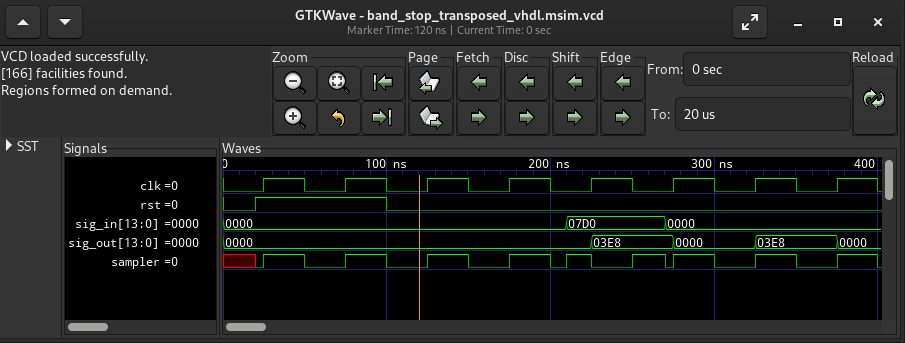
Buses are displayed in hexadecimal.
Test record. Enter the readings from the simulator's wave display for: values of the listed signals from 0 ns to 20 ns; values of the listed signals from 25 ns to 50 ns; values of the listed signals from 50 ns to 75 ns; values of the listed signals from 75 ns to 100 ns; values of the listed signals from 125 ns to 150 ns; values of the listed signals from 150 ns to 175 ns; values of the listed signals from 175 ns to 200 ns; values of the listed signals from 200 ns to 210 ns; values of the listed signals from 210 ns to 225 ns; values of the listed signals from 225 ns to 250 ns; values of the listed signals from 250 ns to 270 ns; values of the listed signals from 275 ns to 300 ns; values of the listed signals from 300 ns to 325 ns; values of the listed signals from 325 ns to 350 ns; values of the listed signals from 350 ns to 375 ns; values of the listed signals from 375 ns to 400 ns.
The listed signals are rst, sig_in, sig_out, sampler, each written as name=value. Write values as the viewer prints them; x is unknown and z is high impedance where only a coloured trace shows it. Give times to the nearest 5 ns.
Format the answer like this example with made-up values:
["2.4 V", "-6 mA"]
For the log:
["rst=0, sig_in=0000, sig_out=0000, sampler=x", "rst=1, sig_in=0000, sig_out=0000, sampler=1", "rst=1, sig_in=0000, sig_out=0000, sampler=0", "rst=1, sig_in=0000, sig_out=0000, sampler=1", "rst=0, sig_in=0000, sig_out=0000, sampler=1", "rst=0, sig_in=0000, sig_out=0000, sampler=0", "rst=0, sig_in=0000, sig_out=0000, sampler=1", "rst=0, sig_in=0000, sig_out=0000, sampler=0", "rst=0, sig_in=07D0, sig_out=0000, sampler=1", "rst=0, sig_in=07D0, sig_out=03E8, sampler=0", "rst=0, sig_in=07D0, sig_out=03E8, sampler=1", "rst=0, sig_in=0000, sig_out=0000, sampler=1", "rst=0, sig_in=0000, sig_out=0000, sampler=0", "rst=0, sig_in=0000, sig_out=03E8, sampler=1", "rst=0, sig_in=0000, sig_out=03E8, sampler=0", "rst=0, sig_in=0000, sig_out=0000, sampler=1"]
